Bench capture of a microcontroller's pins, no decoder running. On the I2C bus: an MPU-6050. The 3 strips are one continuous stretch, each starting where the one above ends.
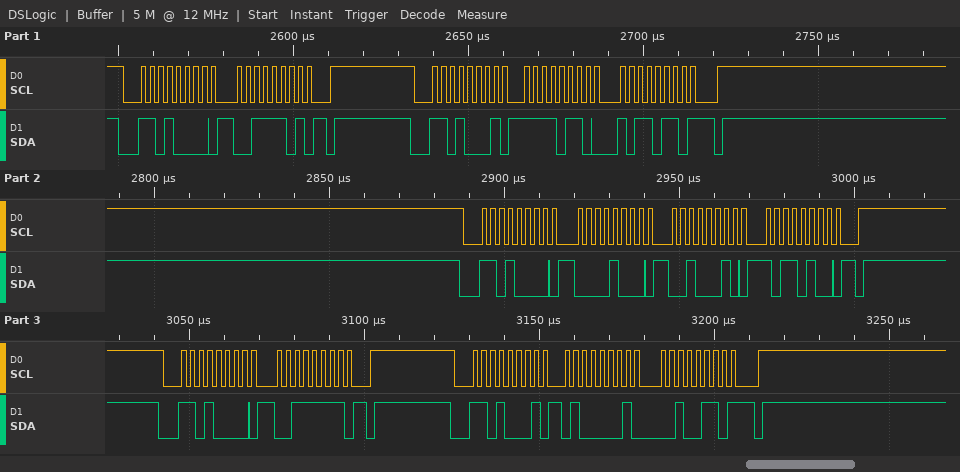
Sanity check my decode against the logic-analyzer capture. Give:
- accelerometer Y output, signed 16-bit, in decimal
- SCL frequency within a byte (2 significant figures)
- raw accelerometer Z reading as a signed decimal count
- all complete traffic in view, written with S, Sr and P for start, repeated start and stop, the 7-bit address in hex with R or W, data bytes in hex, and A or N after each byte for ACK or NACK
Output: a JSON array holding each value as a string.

["-2378", "400 kHz", "16678", "S 68W A 3D A P S 68R A F6 A B6 N P S 68W A 08 A 22 A B4 A P S 68W A 3F A P S 68R A 41 A 26 N P"]
